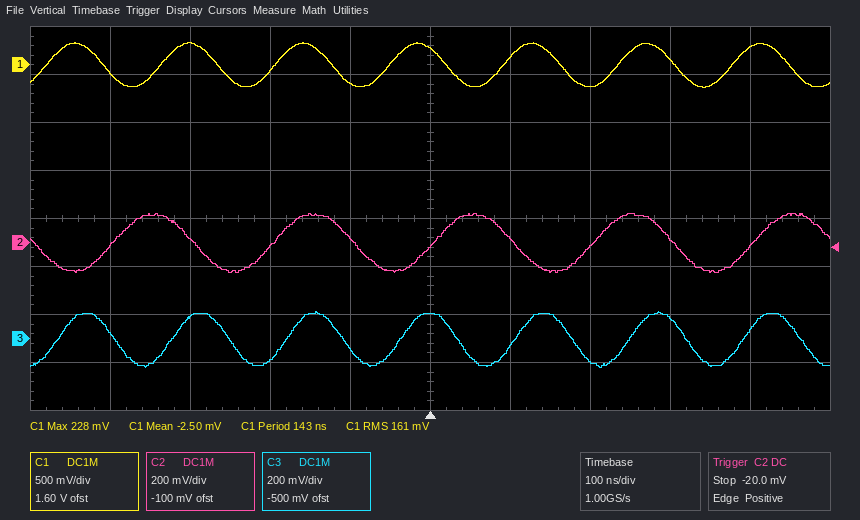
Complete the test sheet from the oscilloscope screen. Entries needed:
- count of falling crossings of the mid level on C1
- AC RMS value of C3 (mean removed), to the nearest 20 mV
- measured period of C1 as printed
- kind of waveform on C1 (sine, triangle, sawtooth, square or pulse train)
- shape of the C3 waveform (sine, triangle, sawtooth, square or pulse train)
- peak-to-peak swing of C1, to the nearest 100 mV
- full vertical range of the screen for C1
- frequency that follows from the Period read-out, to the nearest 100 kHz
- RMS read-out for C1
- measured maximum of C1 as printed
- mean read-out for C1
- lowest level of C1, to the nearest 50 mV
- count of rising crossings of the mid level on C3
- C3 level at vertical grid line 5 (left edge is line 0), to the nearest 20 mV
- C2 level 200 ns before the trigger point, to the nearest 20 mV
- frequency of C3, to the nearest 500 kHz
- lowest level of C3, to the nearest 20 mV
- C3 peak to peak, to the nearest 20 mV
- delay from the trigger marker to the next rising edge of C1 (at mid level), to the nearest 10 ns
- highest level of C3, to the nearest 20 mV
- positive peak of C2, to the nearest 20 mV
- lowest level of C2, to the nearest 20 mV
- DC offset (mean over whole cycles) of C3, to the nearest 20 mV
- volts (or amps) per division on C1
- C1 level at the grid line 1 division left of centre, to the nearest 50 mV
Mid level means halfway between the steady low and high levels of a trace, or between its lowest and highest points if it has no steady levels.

7
80 mV
143 ns
sine
sine
500 mV
4 V
7.0 MHz
161 mV
228 mV
-2.50 mV
-250 mV
7
100 mV
-20 mV
7.0 MHz
-120 mV
240 mV
90 ns
120 mV
120 mV
-120 mV
0 mV
500 mV
-200 mV
